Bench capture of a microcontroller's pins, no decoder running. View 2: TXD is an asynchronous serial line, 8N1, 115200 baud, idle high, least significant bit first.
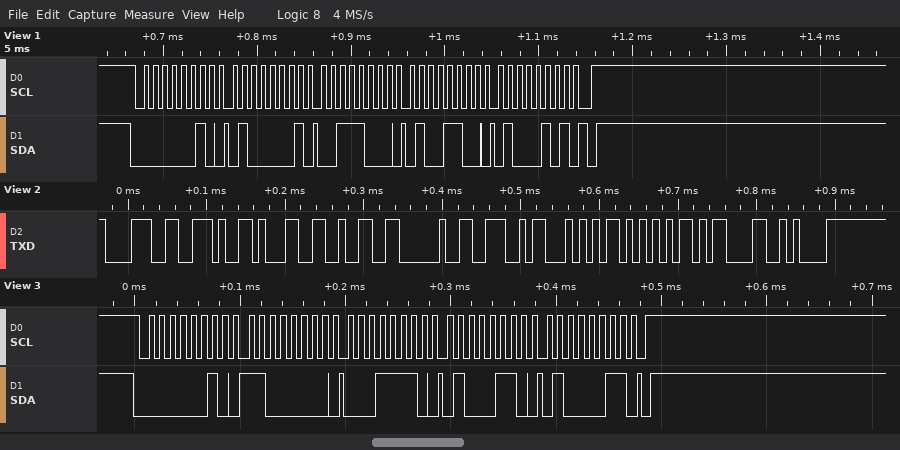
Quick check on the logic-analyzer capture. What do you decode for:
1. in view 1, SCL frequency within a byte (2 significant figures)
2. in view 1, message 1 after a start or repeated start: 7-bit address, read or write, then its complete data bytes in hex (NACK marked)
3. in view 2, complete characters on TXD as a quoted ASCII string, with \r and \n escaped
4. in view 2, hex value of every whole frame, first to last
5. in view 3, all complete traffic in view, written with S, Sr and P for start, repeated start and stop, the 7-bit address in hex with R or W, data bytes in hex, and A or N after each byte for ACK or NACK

100 kHz
0x01 write: 41 38 4C 45
"8.12 NTU\r\n"
38 2E 31 32 20 4E 54 55 0D 0A
S 01W A C0 A 1E A 46 A 43 A P
